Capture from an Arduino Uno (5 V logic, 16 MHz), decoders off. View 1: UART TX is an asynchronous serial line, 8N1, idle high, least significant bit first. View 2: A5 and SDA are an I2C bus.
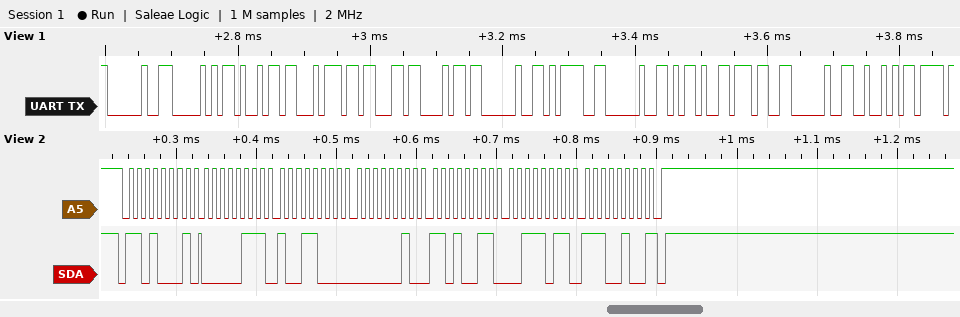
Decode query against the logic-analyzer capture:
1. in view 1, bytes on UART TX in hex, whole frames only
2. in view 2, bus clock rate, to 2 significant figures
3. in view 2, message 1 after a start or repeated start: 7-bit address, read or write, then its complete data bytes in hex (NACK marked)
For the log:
20 50 69 74 63 68 20 3D 20 2D 37 20 52
100 kHz
0x68 read: 07 98 02 D3 3B E4 NACK
